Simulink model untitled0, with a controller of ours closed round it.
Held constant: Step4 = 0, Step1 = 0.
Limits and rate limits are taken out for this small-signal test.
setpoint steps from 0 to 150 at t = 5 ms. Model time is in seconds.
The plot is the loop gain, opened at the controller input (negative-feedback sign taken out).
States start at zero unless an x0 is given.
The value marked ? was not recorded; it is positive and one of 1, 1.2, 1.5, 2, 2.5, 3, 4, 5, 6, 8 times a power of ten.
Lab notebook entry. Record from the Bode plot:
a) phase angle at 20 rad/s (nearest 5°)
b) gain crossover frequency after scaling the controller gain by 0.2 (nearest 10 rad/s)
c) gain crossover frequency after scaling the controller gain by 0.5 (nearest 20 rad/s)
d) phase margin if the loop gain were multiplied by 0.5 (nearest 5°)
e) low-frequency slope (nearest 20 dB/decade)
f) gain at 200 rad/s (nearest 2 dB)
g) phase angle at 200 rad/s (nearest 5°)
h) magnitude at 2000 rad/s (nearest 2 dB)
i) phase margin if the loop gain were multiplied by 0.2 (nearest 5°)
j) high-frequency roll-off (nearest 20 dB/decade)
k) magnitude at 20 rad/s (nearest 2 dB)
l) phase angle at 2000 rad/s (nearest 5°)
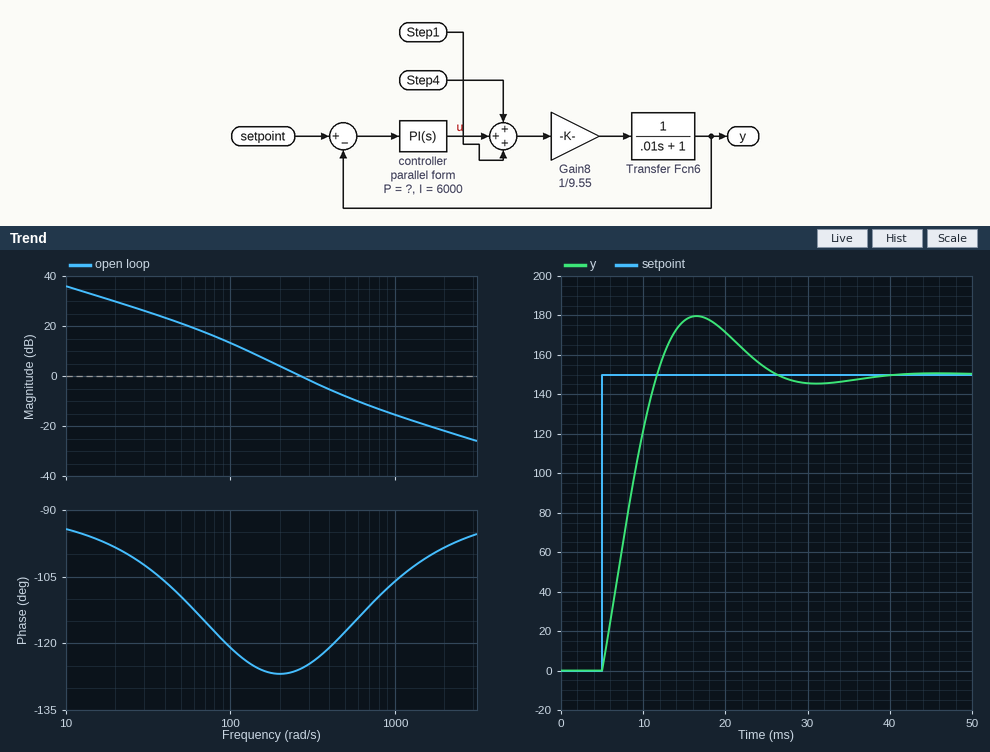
-100°
90 rad/s
180 rad/s
55°
-20 dB/decade
4 dB
-125°
-22 dB
60°
-20 dB/decade
30 dB
-100°
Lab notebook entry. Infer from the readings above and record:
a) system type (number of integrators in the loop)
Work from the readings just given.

1
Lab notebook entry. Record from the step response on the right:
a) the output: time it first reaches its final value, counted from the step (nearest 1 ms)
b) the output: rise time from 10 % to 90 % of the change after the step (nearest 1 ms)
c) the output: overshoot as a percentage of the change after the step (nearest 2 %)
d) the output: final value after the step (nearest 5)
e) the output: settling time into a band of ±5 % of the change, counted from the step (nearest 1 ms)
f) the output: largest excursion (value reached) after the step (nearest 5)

7 ms
5 ms
20 %
150
19 ms
180
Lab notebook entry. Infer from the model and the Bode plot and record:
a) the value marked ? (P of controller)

15
